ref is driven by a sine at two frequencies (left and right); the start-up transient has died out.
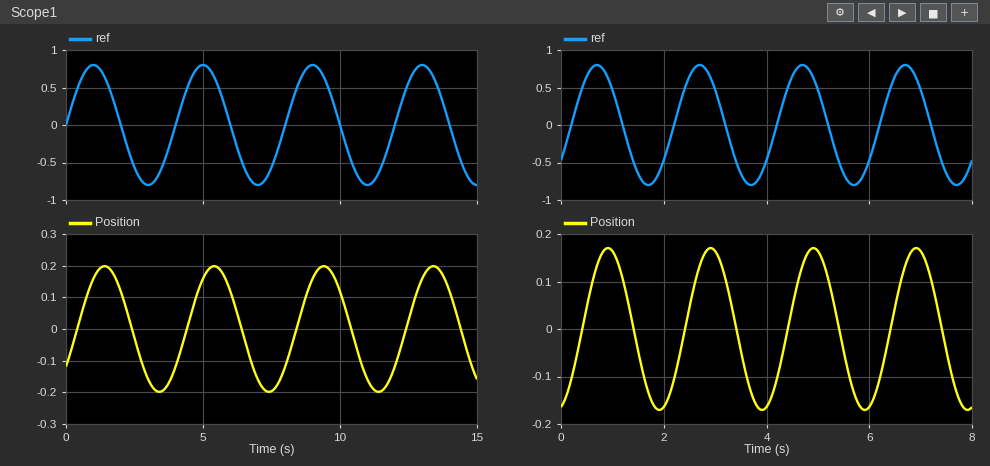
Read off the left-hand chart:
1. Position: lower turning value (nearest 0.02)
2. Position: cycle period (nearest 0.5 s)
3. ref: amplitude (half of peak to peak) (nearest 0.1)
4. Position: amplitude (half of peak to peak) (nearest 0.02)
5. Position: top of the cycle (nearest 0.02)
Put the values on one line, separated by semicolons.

-0.20; 4.0 s; 0.8; 0.20; 0.20
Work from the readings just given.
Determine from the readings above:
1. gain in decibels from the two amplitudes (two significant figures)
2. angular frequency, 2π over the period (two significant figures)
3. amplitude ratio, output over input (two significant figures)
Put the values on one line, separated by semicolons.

-12 dB; 1.6 rad/s; 0.25
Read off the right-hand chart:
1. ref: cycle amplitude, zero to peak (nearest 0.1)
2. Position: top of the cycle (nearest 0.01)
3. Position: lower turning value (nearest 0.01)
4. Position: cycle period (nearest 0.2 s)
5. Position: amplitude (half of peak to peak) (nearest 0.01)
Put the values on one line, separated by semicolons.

0.8; 0.17; -0.17; 2.0 s; 0.17
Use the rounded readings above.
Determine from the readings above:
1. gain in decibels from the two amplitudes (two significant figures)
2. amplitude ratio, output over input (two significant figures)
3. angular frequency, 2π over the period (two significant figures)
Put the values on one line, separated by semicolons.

-13 dB; 0.21; 3.1 rad/s
